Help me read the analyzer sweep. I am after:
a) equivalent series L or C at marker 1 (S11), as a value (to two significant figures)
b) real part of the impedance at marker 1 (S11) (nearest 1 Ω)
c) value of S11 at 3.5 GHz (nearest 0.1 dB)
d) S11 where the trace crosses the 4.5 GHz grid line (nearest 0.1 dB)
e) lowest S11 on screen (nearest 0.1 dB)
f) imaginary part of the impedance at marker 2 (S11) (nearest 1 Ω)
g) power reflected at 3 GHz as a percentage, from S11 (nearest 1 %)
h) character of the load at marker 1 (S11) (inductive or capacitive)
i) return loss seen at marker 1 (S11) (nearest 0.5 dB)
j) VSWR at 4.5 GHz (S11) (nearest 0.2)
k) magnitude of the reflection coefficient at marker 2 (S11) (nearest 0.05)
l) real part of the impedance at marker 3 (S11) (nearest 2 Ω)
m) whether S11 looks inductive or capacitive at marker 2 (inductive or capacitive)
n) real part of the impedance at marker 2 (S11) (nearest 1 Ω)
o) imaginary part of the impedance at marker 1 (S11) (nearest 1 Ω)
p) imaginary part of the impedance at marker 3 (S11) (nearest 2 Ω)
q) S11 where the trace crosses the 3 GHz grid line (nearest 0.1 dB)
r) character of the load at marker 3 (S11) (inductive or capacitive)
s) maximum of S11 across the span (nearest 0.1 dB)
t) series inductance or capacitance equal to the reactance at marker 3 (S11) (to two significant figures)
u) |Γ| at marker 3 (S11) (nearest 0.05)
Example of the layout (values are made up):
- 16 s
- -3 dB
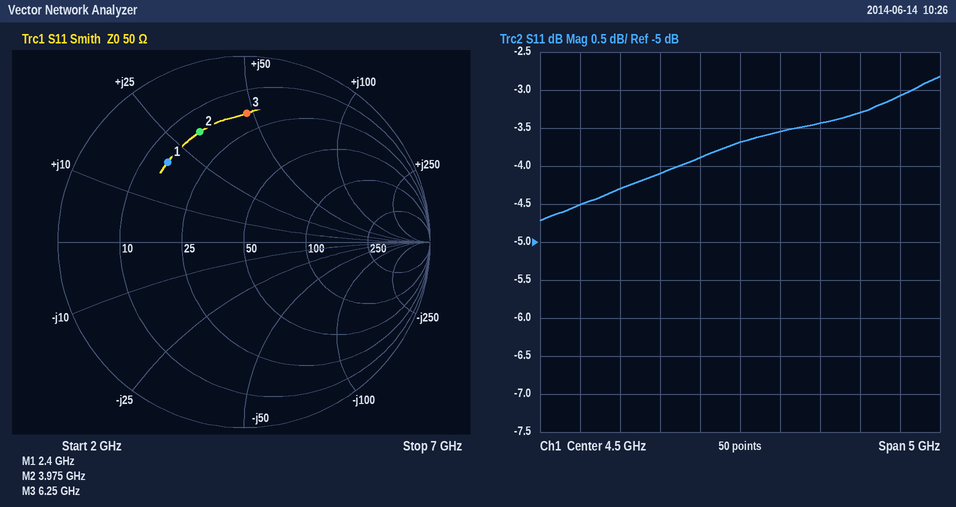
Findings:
- 1.3 nH
- 15 Ω
- -4.1 dB
- -3.7 dB
- -4.7 dB
- +31 Ω
- 37 %
- inductive
- 4.5 dB
- 4.8
- 0.65
- 18 Ω
- inductive
- 16 Ω
- +20 Ω
- +48 Ω
- -4.3 dB
- inductive
- -2.8 dB
- 1.2 nH
- 0.70
